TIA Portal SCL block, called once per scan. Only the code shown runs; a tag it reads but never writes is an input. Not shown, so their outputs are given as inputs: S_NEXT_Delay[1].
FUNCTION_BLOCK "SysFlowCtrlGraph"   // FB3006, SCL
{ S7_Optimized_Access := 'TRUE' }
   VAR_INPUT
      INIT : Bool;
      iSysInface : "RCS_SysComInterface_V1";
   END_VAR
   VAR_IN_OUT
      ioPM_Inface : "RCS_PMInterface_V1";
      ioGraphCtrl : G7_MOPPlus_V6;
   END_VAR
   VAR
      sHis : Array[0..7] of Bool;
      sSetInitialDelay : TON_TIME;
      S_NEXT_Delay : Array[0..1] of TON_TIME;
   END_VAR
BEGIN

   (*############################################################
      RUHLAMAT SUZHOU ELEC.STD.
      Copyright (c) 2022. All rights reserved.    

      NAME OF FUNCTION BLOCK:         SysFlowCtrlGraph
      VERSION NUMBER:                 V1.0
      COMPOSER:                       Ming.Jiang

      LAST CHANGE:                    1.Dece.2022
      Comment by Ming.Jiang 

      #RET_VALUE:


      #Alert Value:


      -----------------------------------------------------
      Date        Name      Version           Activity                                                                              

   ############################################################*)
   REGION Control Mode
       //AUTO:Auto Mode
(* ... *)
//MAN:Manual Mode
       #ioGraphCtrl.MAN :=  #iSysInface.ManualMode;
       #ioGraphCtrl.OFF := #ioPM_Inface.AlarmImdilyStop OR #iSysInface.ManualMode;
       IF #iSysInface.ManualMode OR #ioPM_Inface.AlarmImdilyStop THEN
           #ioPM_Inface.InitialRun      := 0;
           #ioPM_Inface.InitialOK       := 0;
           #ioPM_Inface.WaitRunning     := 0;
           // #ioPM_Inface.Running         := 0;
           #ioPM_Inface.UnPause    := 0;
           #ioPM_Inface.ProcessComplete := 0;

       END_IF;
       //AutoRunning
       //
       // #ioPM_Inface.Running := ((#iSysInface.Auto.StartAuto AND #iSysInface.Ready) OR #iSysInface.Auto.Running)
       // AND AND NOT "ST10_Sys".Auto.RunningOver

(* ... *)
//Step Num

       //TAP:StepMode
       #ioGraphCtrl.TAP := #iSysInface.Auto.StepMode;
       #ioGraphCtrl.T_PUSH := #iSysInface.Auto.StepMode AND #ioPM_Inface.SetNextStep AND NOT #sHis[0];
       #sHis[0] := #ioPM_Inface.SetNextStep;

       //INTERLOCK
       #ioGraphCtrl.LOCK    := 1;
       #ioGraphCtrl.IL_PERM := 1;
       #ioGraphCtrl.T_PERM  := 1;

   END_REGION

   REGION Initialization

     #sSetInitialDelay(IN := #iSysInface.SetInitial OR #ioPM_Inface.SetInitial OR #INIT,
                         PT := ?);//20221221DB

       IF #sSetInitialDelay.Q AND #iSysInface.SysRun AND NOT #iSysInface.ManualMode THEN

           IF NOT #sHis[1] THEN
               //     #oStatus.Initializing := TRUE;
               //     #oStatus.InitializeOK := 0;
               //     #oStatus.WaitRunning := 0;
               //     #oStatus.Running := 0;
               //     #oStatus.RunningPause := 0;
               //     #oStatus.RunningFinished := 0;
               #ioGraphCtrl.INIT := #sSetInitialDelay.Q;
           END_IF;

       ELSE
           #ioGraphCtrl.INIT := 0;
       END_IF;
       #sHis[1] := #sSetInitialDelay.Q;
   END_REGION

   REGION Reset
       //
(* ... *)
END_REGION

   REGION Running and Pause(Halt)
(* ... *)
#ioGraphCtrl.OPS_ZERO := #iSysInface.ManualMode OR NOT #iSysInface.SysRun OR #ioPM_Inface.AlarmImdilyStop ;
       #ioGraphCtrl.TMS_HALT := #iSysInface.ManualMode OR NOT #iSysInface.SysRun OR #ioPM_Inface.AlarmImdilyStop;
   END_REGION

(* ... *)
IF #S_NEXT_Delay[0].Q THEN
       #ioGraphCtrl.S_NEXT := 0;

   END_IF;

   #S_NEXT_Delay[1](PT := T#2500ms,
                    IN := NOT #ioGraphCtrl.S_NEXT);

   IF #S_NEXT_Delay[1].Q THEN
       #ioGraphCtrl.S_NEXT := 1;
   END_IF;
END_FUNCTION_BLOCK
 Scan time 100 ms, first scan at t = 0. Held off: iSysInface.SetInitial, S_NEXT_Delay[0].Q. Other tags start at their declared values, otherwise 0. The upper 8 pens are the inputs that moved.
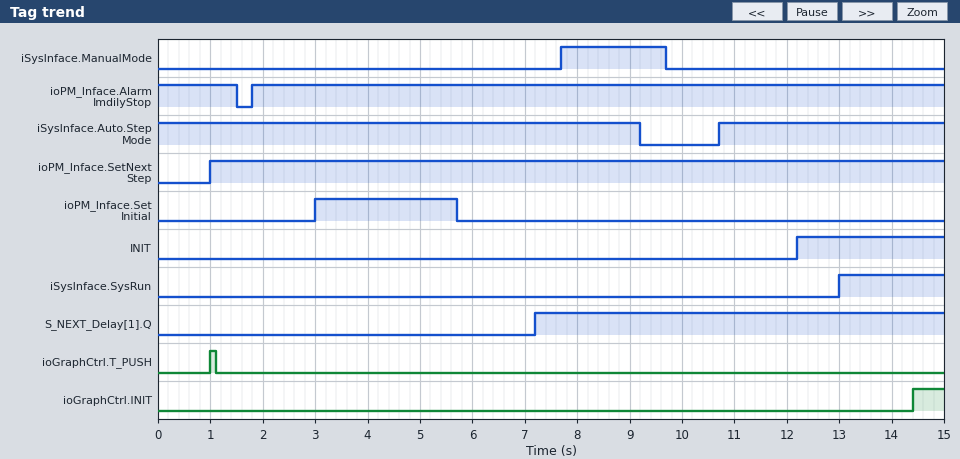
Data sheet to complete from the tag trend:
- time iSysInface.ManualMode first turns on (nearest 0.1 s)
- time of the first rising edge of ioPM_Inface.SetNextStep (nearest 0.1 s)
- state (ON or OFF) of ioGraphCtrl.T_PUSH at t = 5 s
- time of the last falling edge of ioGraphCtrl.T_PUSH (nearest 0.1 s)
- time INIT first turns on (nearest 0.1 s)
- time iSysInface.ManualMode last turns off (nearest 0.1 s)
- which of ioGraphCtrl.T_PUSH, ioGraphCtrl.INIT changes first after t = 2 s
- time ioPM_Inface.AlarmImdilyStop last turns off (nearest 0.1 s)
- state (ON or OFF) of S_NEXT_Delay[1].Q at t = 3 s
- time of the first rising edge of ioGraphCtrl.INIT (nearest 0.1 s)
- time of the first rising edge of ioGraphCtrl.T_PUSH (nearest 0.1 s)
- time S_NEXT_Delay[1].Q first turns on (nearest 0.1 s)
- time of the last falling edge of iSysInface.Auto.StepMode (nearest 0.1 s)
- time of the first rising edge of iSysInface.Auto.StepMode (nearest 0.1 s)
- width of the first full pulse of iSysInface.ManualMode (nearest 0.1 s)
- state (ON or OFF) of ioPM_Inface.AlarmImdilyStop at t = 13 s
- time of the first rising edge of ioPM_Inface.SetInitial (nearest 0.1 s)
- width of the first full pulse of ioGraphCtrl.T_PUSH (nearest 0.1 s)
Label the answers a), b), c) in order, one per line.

a) 7.7 s
b) 1.0 s
c) OFF
d) 1.1 s
e) 12.2 s
f) 9.7 s
g) ioGraphCtrl.INIT
h) 1.5 s
i) OFF
j) 14.4 s
k) 1.0 s
l) 7.2 s
m) 9.2 s
n) 10.7 s
o) 2.0 s
p) ON
q) 3.0 s
r) 0.1 s
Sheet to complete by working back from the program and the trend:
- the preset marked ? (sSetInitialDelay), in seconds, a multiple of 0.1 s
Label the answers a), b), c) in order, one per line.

a) 2.2 s
